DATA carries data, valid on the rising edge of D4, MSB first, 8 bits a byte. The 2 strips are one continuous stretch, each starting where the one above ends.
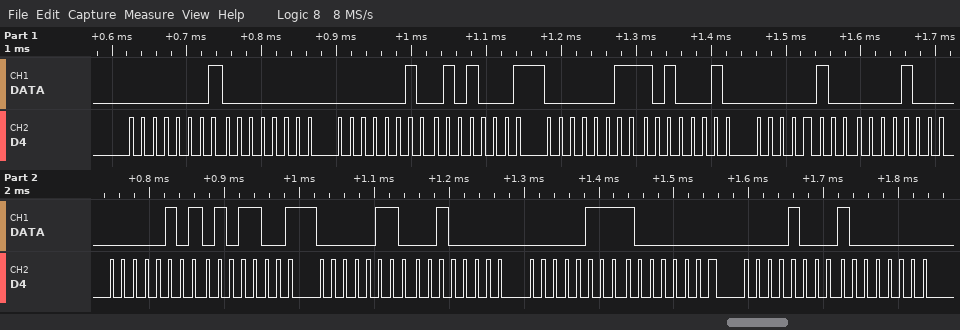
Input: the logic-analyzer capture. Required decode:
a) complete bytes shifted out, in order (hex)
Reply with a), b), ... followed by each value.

a) 01 00 02 51 03 A2 04 08 05 59 06 20 07 80 08 80
